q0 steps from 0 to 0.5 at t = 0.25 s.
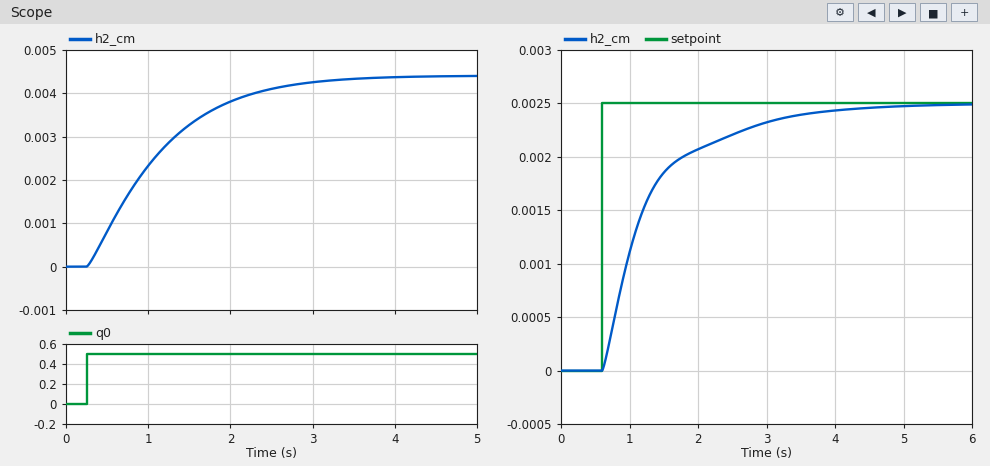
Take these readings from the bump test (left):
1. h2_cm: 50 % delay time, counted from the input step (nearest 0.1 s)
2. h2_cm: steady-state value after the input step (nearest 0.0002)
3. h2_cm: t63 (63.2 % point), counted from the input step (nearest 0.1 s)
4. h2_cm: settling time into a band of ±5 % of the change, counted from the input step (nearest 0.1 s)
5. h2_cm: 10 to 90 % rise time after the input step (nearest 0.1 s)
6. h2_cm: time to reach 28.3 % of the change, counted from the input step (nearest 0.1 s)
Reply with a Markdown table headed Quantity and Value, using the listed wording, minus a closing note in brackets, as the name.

| Quantity | Value |
|---|---|
| h2_cm: 50 % delay time, counted from the input step | 0.7 s |
| h2_cm: steady-state value after the input step | 0.0044 |
| h2_cm: t63 (63.2 % point), counted from the input step | 1.0 s |
| h2_cm: settling time into a band of ±5 % of the change, counted from the input step | 2.5 s |
| h2_cm: 10 to 90 % rise time after the input step | 1.8 s |
| h2_cm: time to reach 28.3 % of the change, counted from the input step | 0.4 s |
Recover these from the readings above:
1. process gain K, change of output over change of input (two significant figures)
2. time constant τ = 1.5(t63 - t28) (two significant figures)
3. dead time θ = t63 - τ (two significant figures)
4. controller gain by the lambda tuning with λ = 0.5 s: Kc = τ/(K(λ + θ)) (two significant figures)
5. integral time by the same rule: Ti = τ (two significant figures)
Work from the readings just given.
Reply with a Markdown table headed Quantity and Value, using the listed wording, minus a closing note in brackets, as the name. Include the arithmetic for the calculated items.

| Quantity | Value |
|---|---|
| process gain K, change of output over change of input | (0.0044 - 0) / 0.5 = 0.0088 |
| time constant τ = 1.5(t63 - t28) | 1.5 × (1 - 0.4) = 0.90 s |
| dead time θ = t63 - τ | 1 - 0.9 = 0.10 s |
| controller gain by the lambda tuning with λ = 0.5 s: Kc = τ/(K(λ + θ)) | 0.9 / (0.0088 × (0.5 + 0.1)) = 170 |
| integral time by the same rule: Ti = τ | 0.90 s |
